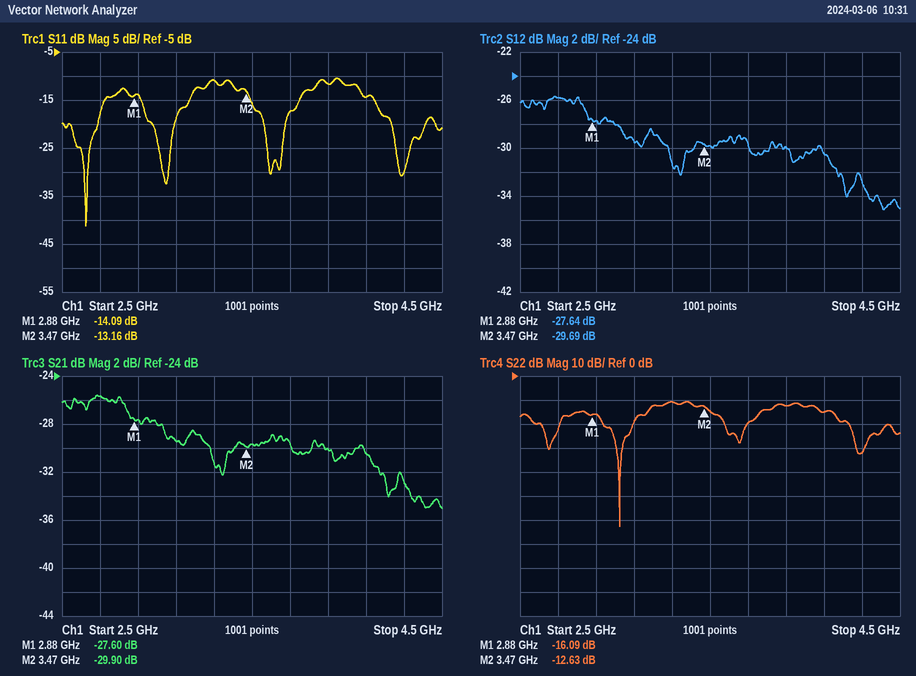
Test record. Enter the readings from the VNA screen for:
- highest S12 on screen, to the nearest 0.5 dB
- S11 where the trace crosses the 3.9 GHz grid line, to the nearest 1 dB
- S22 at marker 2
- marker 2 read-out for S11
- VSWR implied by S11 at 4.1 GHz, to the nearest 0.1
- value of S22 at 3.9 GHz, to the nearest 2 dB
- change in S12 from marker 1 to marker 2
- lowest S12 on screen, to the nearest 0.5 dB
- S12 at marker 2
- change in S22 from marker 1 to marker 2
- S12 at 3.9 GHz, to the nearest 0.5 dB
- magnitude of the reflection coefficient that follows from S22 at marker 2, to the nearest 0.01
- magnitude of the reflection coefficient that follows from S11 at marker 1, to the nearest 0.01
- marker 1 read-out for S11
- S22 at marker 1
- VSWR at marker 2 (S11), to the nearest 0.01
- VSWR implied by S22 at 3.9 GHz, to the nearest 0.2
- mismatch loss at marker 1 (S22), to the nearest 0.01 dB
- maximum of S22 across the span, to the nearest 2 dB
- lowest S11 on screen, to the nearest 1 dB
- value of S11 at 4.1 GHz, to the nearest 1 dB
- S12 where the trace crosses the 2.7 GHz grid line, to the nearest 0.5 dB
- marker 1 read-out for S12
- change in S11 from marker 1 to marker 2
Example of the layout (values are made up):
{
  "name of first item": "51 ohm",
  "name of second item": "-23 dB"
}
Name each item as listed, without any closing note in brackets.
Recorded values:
{
  "highest S12 on screen, to the nearest 0.5 dB": "-25.5 dB",
  "S11 where the trace crosses the 3.9 GHz grid line, to the nearest 1 dB": "-12 dB",
  "S22 at marker 2": "-12.63 dB",
  "marker 2 read-out for S11": "-13.16 dB",
  "VSWR implied by S11 at 4.1 GHz, to the nearest 0.1": "1.5",
  "value of S22 at 3.9 GHz, to the nearest 2 dB": "-12 dB",
  "change in S12 from marker 1 to marker 2": "-2.05 dB",
  "lowest S12 on screen, to the nearest 0.5 dB": "-35.0 dB",
  "S12 at marker 2": "-29.69 dB",
  "change in S22 from marker 1 to marker 2": "3.46 dB",
  "S12 at 3.9 GHz, to the nearest 0.5 dB": "-30.0 dB",
  "magnitude of the reflection coefficient that follows from S22 at marker 2, to the nearest 0.01": "0.23",
  "magnitude of the reflection coefficient that follows from S11 at marker 1, to the nearest 0.01": "0.20",
  "marker 1 read-out for S11": "-14.09 dB",
  "S22 at marker 1": "-16.09 dB",
  "VSWR at marker 2 (S11), to the nearest 0.01": "1.56",
  "VSWR implied by S22 at 3.9 GHz, to the nearest 0.2": "1.6",
  "mismatch loss at marker 1 (S22), to the nearest 0.01 dB": "0.11 dB",
  "maximum of S22 across the span, to the nearest 2 dB": "-10 dB",
  "lowest S11 on screen, to the nearest 1 dB": "-41 dB",
  "value of S11 at 4.1 GHz, to the nearest 1 dB": "-14 dB",
  "S12 where the trace crosses the 2.7 GHz grid line, to the nearest 0.5 dB": "-26.0 dB",
  "marker 1 read-out for S12": "-27.64 dB",
  "change in S11 from marker 1 to marker 2": "0.93 dB"
}
